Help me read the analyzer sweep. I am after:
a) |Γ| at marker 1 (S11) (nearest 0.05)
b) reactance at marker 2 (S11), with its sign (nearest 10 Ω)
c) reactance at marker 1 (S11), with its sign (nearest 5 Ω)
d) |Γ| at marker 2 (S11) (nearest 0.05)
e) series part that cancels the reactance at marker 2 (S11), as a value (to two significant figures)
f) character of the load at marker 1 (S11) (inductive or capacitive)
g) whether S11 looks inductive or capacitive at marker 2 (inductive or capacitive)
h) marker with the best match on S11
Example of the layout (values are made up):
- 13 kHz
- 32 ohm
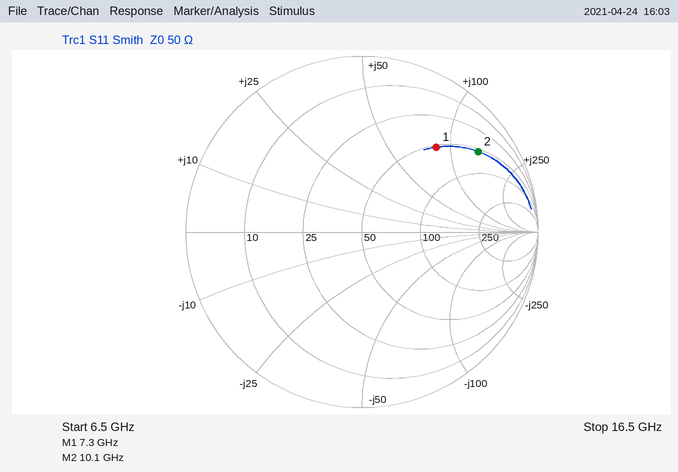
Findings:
- 0.65
- +140 Ω
- +85 Ω
- 0.80
- 110 fF
- inductive
- inductive
- marker 1
